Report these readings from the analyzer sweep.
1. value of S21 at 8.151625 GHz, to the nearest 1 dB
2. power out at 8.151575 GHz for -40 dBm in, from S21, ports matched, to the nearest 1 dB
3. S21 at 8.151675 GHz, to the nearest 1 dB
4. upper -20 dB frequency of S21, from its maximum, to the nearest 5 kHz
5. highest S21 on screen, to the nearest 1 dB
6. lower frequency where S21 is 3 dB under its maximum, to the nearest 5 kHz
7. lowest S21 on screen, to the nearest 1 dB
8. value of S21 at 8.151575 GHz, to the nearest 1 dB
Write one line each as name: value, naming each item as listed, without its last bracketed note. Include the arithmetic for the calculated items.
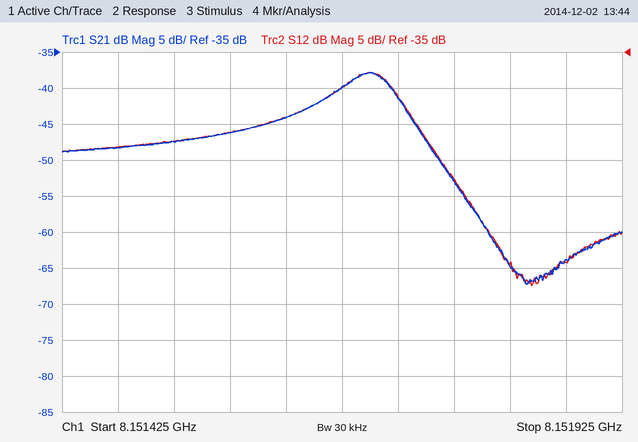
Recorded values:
value of S21 at 8.151625 GHz, to the nearest 1 dB: -44 dB
power out at 8.151575 GHz for -40 dBm in, from S21, ports matched, to the nearest 1 dB: -40 dBm + (-46 dB) = -86 dBm
S21 at 8.151675 GHz, to the nearest 1 dB: -40 dB
upper -20 dB frequency of S21, from its maximum, to the nearest 5 kHz: 8.151795 GHz
highest S21 on screen, to the nearest 1 dB: -38 dB
lower frequency where S21 is 3 dB under its maximum, to the nearest 5 kHz: 8.151665 GHz
lowest S21 on screen, to the nearest 1 dB: -67 dB
value of S21 at 8.151575 GHz, to the nearest 1 dB: -46 dB
